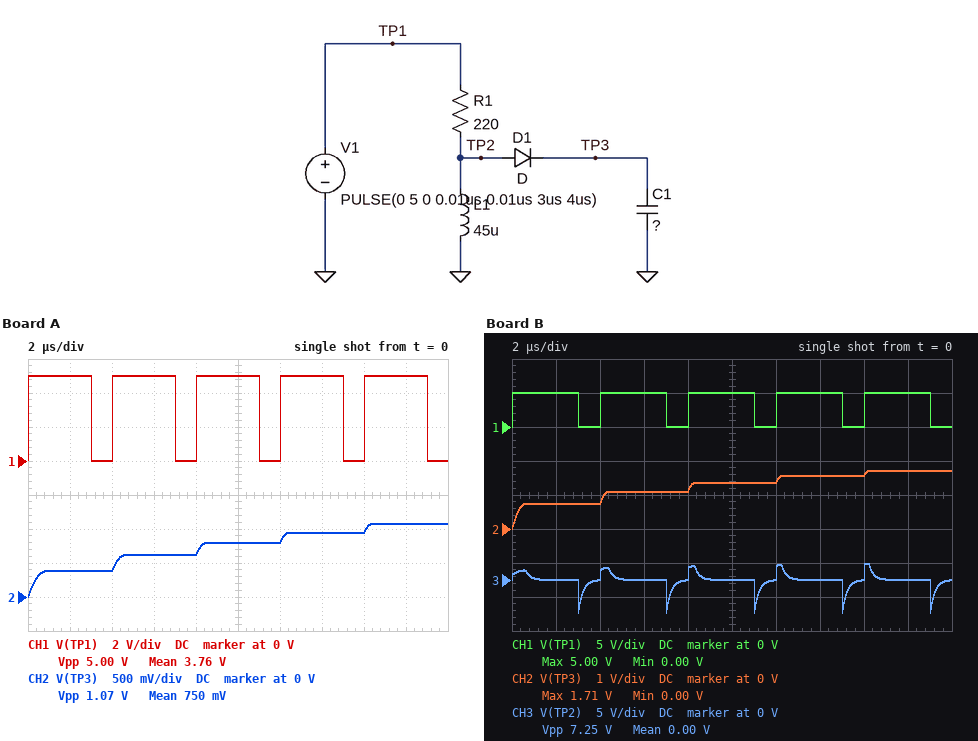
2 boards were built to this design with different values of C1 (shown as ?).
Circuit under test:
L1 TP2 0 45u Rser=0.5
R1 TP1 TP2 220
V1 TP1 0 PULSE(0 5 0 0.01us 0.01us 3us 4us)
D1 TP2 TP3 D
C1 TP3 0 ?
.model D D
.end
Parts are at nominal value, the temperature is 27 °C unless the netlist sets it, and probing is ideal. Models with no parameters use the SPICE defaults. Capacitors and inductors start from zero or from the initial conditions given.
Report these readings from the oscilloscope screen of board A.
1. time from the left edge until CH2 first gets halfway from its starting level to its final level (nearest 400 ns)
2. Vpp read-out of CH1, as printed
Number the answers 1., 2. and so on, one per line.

1. 4.4 µs
2. 5.00 V
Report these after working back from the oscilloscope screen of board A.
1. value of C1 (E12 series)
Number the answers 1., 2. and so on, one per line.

1. 22 nF
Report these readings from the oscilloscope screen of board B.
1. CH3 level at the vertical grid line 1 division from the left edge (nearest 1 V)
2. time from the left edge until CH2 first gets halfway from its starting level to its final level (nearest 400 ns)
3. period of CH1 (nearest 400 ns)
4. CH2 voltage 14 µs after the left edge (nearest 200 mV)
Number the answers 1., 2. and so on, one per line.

1. 0 V
2. 4.0 µs
3. 4.0 µs
4. 1.6 V
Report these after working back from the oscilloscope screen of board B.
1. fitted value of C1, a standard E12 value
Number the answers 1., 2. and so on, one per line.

1. 8.2 nF
